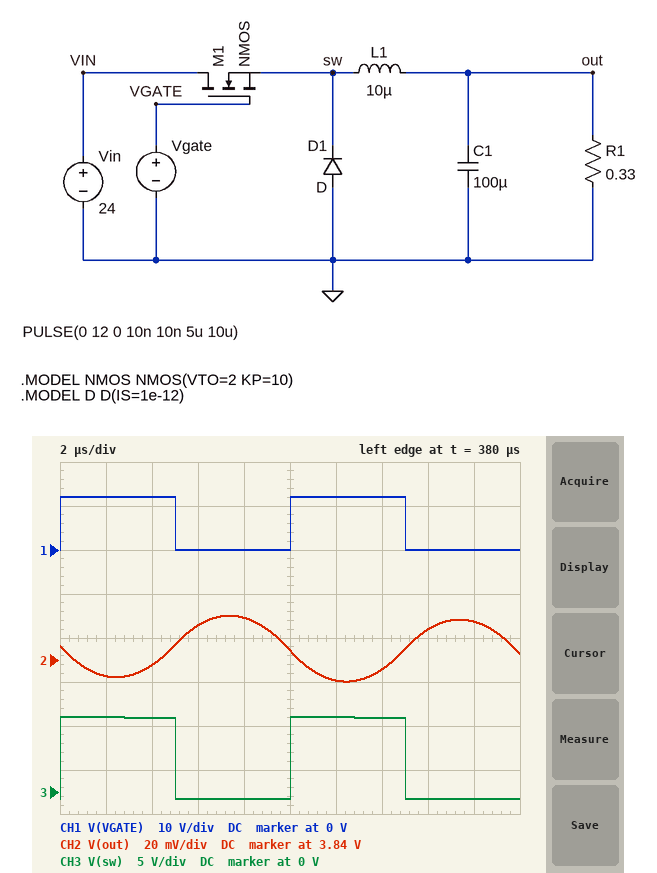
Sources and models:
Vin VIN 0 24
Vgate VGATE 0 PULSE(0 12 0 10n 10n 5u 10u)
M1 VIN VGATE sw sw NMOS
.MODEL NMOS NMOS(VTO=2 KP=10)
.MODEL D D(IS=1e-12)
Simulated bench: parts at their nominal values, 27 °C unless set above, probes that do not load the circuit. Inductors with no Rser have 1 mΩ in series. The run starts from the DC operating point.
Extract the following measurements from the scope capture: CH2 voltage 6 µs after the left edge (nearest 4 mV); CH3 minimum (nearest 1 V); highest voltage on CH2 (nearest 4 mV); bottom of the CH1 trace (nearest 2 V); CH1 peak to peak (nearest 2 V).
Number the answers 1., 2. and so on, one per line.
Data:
1. 3.856 V
2. -1 V
3. 3.860 V
4. 0 V
5. 12 V
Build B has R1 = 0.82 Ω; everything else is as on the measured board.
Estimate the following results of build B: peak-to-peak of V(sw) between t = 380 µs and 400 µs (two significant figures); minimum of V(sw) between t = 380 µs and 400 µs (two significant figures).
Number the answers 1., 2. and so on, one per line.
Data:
1. 9.9 V
2. -760 mV
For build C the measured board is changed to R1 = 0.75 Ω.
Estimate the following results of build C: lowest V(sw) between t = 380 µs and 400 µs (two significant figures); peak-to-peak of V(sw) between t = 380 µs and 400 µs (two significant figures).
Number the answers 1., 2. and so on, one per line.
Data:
1. -760 mV
2. 9.9 V
